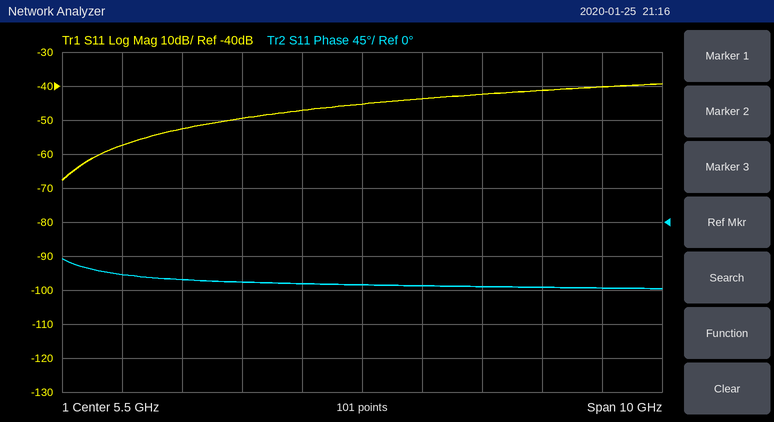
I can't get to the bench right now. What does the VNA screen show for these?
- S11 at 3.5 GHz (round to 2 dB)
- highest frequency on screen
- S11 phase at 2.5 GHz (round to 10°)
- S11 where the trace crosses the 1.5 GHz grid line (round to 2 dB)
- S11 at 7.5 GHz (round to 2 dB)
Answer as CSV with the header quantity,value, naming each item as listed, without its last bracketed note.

quantity,value
S11 at 3.5 GHz,-50 dB
highest frequency on screen,10.5 GHz
S11 phase at 2.5 GHz,-80°
S11 where the trace crosses the 1.5 GHz grid line,-58 dB
S11 at 7.5 GHz,-42 dB
